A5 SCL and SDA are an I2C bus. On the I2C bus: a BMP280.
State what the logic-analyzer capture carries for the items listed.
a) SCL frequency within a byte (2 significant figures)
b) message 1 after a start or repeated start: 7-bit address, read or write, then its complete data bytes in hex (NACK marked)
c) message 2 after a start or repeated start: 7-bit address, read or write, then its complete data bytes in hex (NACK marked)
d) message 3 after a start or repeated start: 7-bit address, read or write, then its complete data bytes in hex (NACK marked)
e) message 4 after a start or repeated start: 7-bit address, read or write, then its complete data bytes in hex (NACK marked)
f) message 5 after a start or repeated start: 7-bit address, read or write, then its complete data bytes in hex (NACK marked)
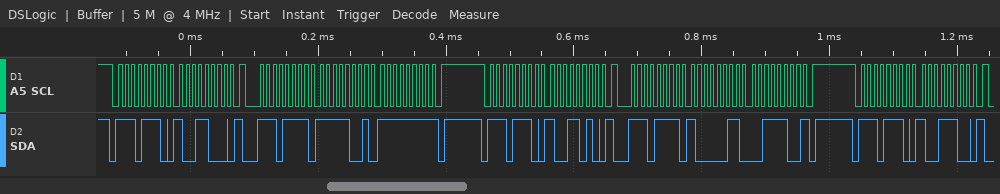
100 kHz
0x77 write: 98
0x77 read: F9 FF NACK
0x77 write: 9A
0x77 read: 83 3C NACK
0x77 write: 9C
